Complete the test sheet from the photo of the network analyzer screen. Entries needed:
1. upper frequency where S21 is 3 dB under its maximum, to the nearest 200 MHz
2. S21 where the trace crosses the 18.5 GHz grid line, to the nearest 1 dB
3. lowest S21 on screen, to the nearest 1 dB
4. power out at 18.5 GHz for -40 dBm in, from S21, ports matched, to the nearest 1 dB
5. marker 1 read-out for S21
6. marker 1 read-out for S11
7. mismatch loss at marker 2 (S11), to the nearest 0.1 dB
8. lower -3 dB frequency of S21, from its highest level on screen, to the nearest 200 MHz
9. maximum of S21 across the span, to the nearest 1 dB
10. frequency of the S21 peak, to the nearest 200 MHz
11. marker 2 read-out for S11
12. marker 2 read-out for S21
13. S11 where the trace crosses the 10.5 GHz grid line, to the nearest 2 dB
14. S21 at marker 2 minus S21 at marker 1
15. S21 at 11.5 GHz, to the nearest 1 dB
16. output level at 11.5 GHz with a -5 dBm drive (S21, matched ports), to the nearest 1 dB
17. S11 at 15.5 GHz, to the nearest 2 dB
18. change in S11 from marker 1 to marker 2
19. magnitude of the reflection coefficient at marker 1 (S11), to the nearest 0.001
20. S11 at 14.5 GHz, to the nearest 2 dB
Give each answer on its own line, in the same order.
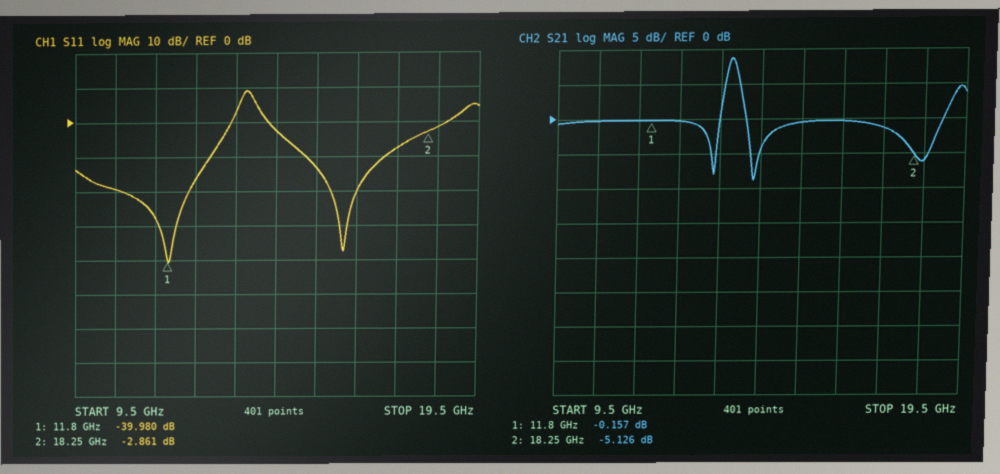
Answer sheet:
14.0 GHz
-6 dB
-9 dB
-46 dBm
-0.157 dB
-39.980 dB
3.2 dB
13.6 GHz
9 dB
13.8 GHz
-2.861 dB
-5.126 dB
-20 dB
-4.969 dB
0 dB
-5 dBm
-14 dB
37.119 dB
0.010
-2 dB
